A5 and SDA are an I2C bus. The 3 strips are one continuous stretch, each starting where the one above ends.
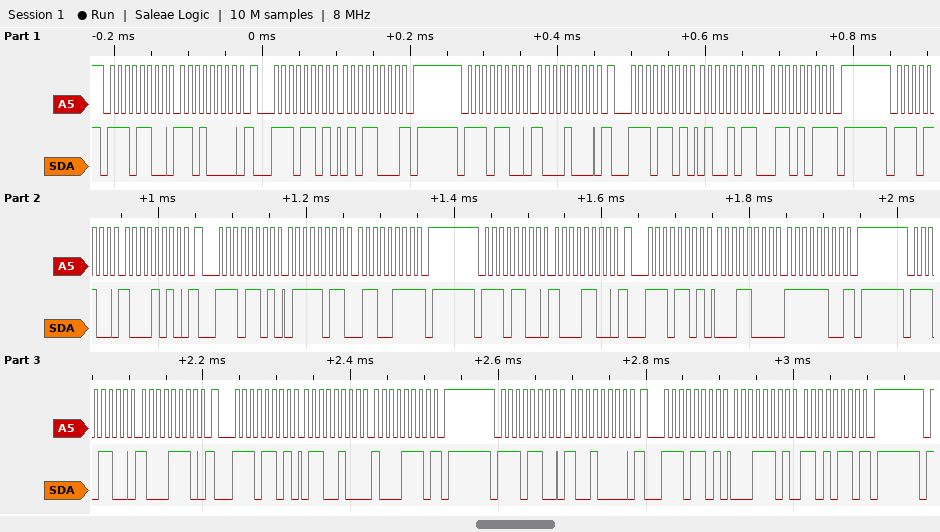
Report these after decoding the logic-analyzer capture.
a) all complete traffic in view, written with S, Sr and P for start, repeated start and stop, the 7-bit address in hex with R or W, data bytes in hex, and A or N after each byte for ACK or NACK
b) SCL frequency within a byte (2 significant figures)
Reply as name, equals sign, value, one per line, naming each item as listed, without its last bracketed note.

all complete traffic in view, written with S, Sr and P for start, repeated start and stop, the 7-bit address in hex with R or W, data bytes in hex, and A or N after each byte for ACK or NACK = S 76W A D0 A Sr 76R A 58 N P S 76W A 88 A Sr 76R A 4B A 6B N P S 76W A 8A A Sr 76R A 7B A 67 N P S 76W A 8C A Sr 76R A 18 A FC N P S 76W A 8E A Sr 76R A 64 A 8E N P S 76W A 90 A Sr 76R A 1D A D6 N P
SCL frequency within a byte = 100 kHz
